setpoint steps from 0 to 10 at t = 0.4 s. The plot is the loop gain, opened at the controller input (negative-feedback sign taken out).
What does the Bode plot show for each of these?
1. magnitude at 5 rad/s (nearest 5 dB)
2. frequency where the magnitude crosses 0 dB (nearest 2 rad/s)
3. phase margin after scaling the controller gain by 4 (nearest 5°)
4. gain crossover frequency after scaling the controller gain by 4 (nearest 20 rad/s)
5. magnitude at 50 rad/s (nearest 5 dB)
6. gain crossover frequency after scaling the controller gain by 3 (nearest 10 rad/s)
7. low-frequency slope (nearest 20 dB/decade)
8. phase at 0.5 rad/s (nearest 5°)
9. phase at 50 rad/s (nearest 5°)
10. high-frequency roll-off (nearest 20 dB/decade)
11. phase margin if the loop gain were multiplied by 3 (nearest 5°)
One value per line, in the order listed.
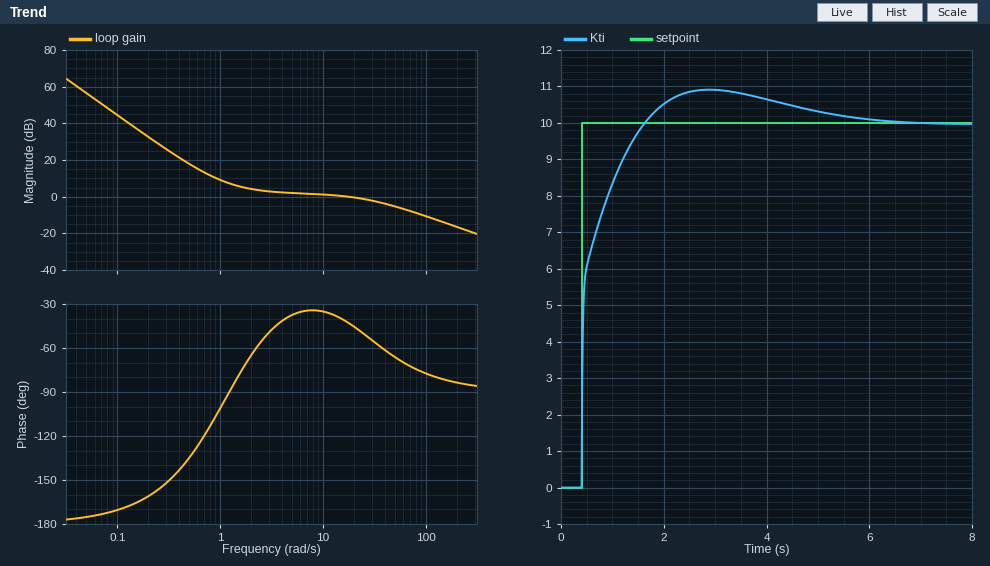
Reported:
0 dB
18 rad/s
100°
120 rad/s
-5 dB
90 rad/s
-40 dB/decade
-135°
-65°
-20 dB/decade
105°
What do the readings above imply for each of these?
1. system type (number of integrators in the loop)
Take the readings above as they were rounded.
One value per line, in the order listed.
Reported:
2
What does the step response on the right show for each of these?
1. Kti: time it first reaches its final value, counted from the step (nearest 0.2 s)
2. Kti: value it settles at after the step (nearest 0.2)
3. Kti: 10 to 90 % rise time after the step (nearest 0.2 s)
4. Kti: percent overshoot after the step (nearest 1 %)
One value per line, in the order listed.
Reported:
1.2 s
10.0
0.8 s
9 %
